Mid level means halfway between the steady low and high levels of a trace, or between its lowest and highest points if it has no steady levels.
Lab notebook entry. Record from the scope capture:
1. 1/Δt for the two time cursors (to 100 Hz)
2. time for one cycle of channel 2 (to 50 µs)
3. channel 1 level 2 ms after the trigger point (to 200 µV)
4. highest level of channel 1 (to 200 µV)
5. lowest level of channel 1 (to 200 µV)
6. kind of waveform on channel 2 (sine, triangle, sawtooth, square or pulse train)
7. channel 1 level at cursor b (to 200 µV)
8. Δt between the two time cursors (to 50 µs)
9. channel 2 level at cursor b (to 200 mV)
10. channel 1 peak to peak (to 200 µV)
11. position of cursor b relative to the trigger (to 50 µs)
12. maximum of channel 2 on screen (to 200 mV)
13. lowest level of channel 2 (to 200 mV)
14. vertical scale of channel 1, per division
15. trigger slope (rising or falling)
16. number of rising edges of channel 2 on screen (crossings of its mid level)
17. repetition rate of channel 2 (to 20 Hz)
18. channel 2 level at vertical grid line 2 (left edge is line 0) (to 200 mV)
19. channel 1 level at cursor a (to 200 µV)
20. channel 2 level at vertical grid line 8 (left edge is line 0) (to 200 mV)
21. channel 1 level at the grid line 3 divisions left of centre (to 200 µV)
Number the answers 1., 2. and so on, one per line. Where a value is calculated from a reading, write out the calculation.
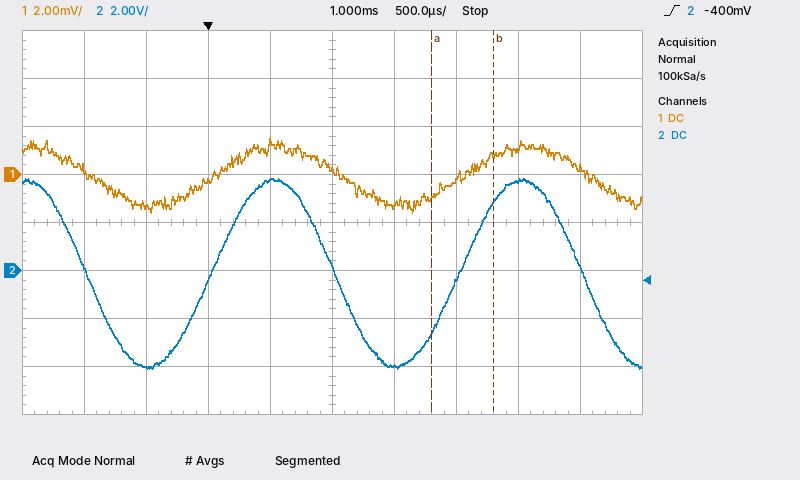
1. 1 / 500 µs ≈ 2.0 kHz
2. 2.00 ms
3. -200 µV
4. 1.6 mV
5. -1.6 mV
6. sine
7. 800 µV
8. 500 µs
9. 2.8 V
10. 1.6 mV − (-1.6 mV) = 3.2 mV
11. +2.30 ms
12. 3.8 V
13. -4.0 V
14. 2 mV
15. rising
16. 2
17. 1 / 2.00 ms ≈ 500 Hz
18. -4.0 V
19. -1.0 mV
20. 3.8 V
21. -1.2 mV
